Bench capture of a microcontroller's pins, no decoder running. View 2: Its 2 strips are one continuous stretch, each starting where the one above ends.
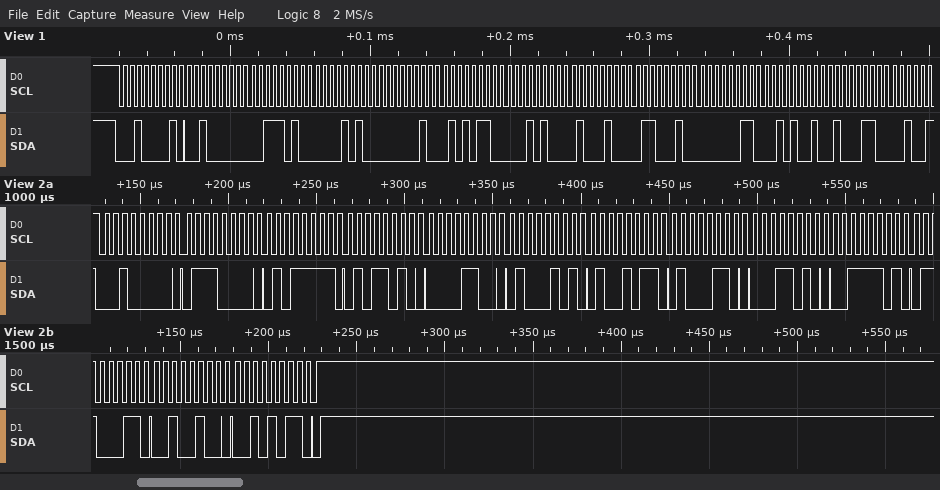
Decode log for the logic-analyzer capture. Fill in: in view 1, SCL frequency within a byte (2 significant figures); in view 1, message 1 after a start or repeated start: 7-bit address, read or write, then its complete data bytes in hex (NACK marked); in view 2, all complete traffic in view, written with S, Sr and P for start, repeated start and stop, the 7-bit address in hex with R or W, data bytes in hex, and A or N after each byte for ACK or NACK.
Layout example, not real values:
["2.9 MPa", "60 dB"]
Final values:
["200 kHz", "0x10 read: 20 3A 0A 02 56 14 44 62 03 29 46", "S 10W A 70 A 5F A 5A A 0C A 45 A 4B A 46 A 1A A 3D A 63 A 24 A 2B A P"]
